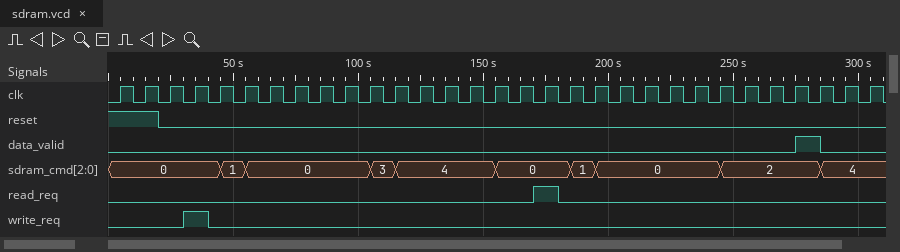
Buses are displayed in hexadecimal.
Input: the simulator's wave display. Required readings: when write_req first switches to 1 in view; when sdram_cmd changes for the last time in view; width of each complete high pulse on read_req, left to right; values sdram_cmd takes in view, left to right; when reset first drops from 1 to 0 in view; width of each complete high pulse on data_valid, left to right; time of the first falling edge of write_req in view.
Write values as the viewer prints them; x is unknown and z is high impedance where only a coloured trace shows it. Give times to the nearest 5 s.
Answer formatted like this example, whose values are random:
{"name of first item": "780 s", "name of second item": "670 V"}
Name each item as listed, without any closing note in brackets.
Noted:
{"when write_req first switches to 1 in view": "30 s", "when sdram_cmd changes for the last time in view": "285 s", "width of each complete high pulse on read_req, left to right": "10 s", "values sdram_cmd takes in view, left to right": "0, 1, 0, 3, 4, 0, 1, 0, 2, 4", "when reset first drops from 1 to 0 in view": "20 s", "width of each complete high pulse on data_valid, left to right": "10 s", "time of the first falling edge of write_req in view": "40 s"}
